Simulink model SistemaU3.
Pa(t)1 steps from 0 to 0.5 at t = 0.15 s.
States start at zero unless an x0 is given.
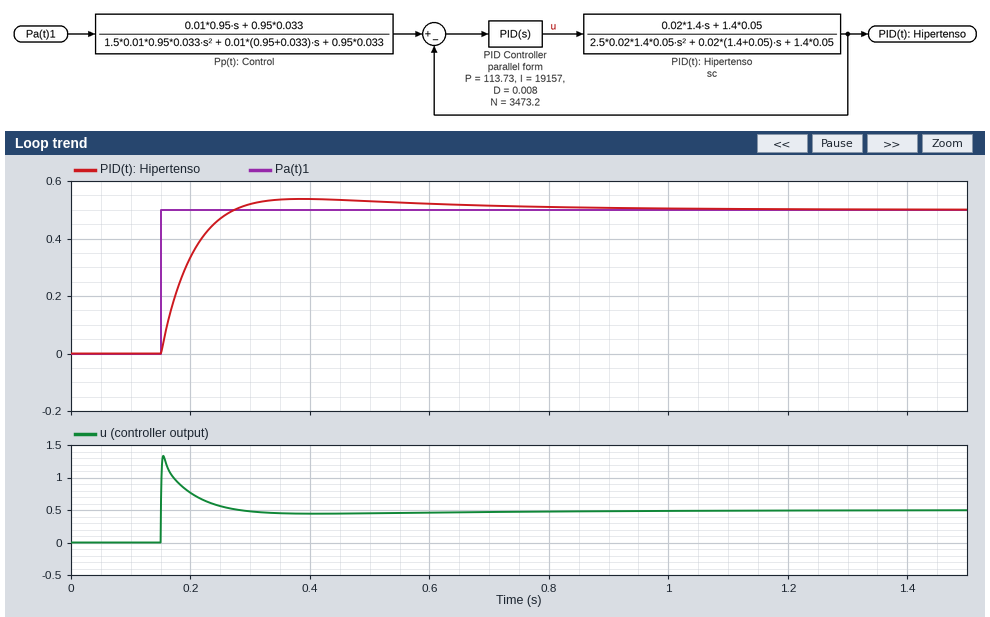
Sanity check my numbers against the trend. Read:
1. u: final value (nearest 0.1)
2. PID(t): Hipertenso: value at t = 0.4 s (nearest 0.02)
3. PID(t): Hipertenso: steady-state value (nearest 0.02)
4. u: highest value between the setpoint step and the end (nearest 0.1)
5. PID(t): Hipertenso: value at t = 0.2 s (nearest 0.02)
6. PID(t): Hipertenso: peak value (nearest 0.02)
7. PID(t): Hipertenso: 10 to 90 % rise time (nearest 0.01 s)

0.5
0.54
0.50
1.3
0.34
0.54
0.08 s
